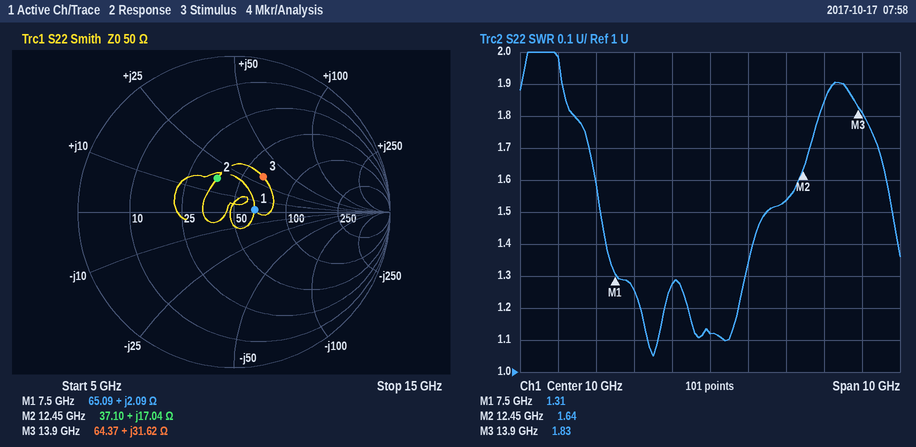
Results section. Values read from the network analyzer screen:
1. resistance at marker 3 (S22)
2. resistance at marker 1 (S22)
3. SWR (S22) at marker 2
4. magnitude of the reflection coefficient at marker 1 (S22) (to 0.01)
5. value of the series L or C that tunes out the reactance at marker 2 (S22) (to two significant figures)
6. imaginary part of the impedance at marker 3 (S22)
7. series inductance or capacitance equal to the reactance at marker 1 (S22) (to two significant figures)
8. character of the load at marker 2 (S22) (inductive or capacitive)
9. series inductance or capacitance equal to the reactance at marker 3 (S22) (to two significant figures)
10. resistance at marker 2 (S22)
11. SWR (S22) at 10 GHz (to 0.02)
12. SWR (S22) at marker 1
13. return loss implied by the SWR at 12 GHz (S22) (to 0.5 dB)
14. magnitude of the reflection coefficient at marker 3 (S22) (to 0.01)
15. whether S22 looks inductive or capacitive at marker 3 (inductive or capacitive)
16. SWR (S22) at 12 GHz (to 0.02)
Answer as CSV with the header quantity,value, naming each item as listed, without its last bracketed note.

quantity,value
resistance at marker 3,64.37 Ω
resistance at marker 1,65.09 Ω
SWR (S22) at marker 2,1.64
magnitude of the reflection coefficient at marker 1 (S22),0.13
value of the series L or C that tunes out the reactance at marker 2 (S22),750 fF
imaginary part of the impedance at marker 3,+31.62 Ω
series inductance or capacitance equal to the reactance at marker 1 (S22),44 pH
character of the load at marker 2 (S22),inductive
series inductance or capacitance equal to the reactance at marker 3 (S22),360 pH
resistance at marker 2,37.10 Ω
SWR (S22) at 10 GHz,1.12
SWR (S22) at marker 1,1.31
return loss implied by the SWR at 12 GHz (S22),13.5 dB
magnitude of the reflection coefficient at marker 3 (S22),0.29
whether S22 looks inductive or capacitive at marker 3,inductive
SWR (S22) at 12 GHz,1.54
